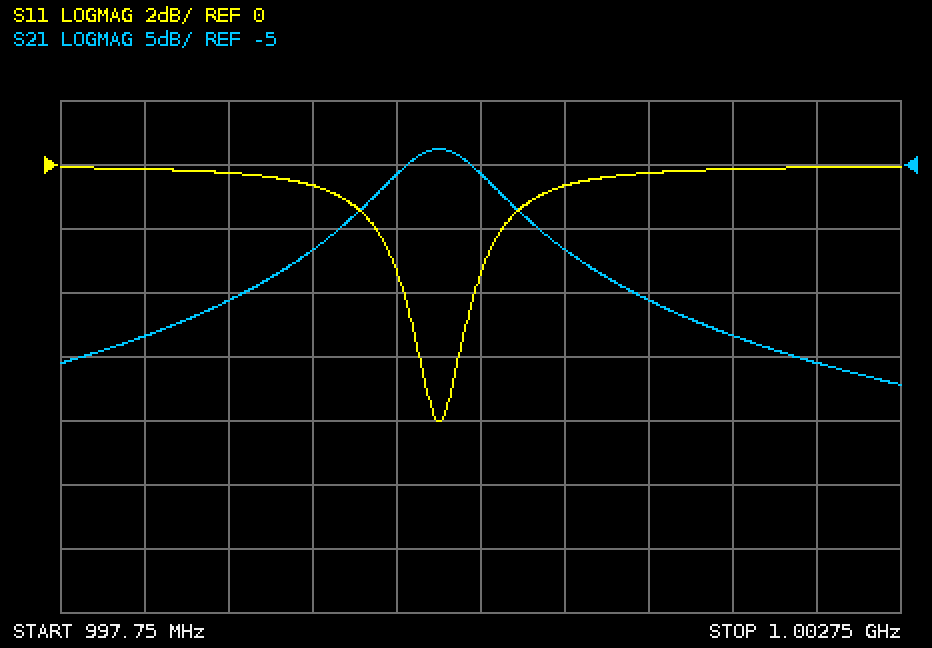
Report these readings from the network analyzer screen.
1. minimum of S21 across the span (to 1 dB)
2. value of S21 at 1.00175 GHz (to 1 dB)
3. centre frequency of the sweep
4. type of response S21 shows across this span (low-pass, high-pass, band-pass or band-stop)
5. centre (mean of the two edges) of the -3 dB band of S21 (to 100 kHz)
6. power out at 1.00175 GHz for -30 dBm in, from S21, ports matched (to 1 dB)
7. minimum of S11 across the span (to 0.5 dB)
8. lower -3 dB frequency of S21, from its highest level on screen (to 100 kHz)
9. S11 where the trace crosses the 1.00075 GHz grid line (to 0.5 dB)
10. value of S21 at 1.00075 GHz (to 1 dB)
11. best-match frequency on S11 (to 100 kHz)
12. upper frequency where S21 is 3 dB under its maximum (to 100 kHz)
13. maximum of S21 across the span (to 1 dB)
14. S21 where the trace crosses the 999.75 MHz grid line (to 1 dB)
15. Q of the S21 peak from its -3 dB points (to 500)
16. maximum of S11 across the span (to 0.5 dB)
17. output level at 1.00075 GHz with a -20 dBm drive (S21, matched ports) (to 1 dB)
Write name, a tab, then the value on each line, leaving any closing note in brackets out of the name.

minimum of S21 across the span	-22 dB
value of S21 at 1.00175 GHz	-18 dB
centre frequency of the sweep	1.00025 GHz
type of response S21 shows across this span	band-pass
centre (mean of the two edges) of the -3 dB band of S21	1.0000 GHz
power out at 1.00175 GHz for -30 dBm in, from S21, ports matched	-48 dBm
minimum of S11 across the span	-8.0 dB
lower -3 dB frequency of S21, from its highest level on screen	999.7 MHz
S11 where the trace crosses the 1.00075 GHz grid line	-0.5 dB
value of S21 at 1.00075 GHz	-12 dB
best-match frequency on S11	1.0000 GHz
upper frequency where S21 is 3 dB under its maximum	1.0003 GHz
maximum of S21 across the span	-4 dB
S21 where the trace crosses the 999.75 MHz grid line	-6 dB
Q of the S21 peak from its -3 dB points	1500
maximum of S11 across the span	0.0 dB
output level at 1.00075 GHz with a -20 dBm drive (S21, matched ports)	-32 dBm
